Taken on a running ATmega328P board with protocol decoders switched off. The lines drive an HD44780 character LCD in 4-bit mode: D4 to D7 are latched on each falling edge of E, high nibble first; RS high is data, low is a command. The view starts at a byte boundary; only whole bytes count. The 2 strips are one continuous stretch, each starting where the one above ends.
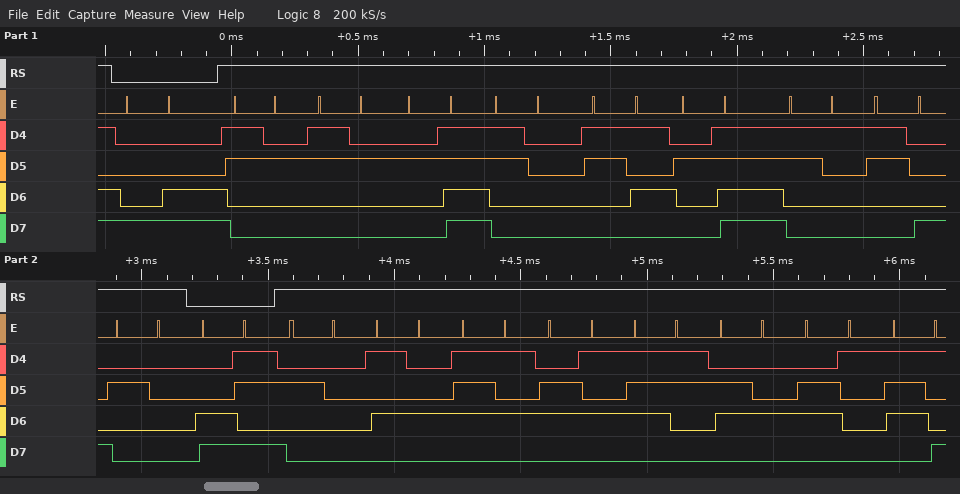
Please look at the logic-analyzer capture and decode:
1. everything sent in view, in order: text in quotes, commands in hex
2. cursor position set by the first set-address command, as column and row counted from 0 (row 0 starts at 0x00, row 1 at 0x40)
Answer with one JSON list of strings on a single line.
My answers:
["0x8C \"22/05/18 \" 0xCB \" Tuesday\"", "column 12, row 0"]
